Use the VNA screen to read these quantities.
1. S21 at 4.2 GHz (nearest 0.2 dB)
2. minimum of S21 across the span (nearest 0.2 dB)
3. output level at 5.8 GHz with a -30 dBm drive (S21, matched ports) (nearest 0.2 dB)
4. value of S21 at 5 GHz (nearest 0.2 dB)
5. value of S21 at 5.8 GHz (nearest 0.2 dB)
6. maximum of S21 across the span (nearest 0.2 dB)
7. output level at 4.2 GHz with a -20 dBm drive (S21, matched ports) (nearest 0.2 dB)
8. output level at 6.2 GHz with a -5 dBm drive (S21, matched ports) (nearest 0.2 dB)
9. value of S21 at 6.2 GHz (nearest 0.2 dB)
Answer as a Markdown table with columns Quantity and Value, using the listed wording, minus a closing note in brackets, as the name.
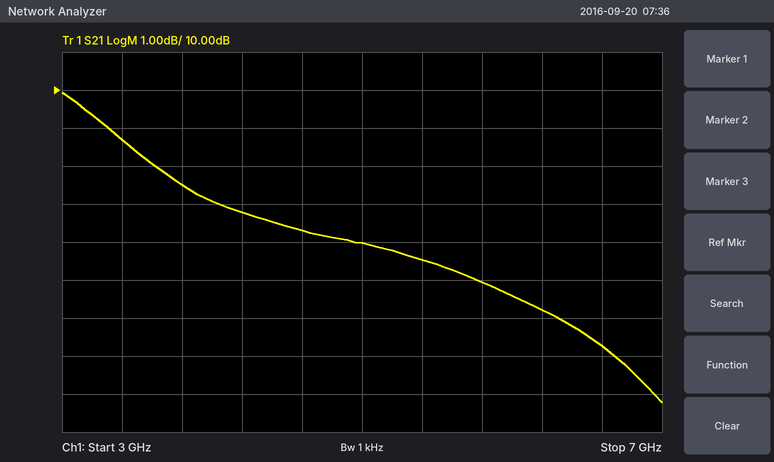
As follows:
| Quantity | Value |
|---|---|
| S21 at 4.2 GHz | 6.8 dB |
| minimum of S21 across the span | 1.8 dB |
| output level at 5.8 GHz with a -30 dBm drive (S21, matched ports) | -25.0 dBm |
| value of S21 at 5 GHz | 6.0 dB |
| value of S21 at 5.8 GHz | 5.0 dB |
| maximum of S21 across the span | 10.0 dB |
| output level at 4.2 GHz with a -20 dBm drive (S21, matched ports) | -13.2 dBm |
| output level at 6.2 GHz with a -5 dBm drive (S21, matched ports) | -0.8 dBm |
| value of S21 at 6.2 GHz | 4.2 dB |
